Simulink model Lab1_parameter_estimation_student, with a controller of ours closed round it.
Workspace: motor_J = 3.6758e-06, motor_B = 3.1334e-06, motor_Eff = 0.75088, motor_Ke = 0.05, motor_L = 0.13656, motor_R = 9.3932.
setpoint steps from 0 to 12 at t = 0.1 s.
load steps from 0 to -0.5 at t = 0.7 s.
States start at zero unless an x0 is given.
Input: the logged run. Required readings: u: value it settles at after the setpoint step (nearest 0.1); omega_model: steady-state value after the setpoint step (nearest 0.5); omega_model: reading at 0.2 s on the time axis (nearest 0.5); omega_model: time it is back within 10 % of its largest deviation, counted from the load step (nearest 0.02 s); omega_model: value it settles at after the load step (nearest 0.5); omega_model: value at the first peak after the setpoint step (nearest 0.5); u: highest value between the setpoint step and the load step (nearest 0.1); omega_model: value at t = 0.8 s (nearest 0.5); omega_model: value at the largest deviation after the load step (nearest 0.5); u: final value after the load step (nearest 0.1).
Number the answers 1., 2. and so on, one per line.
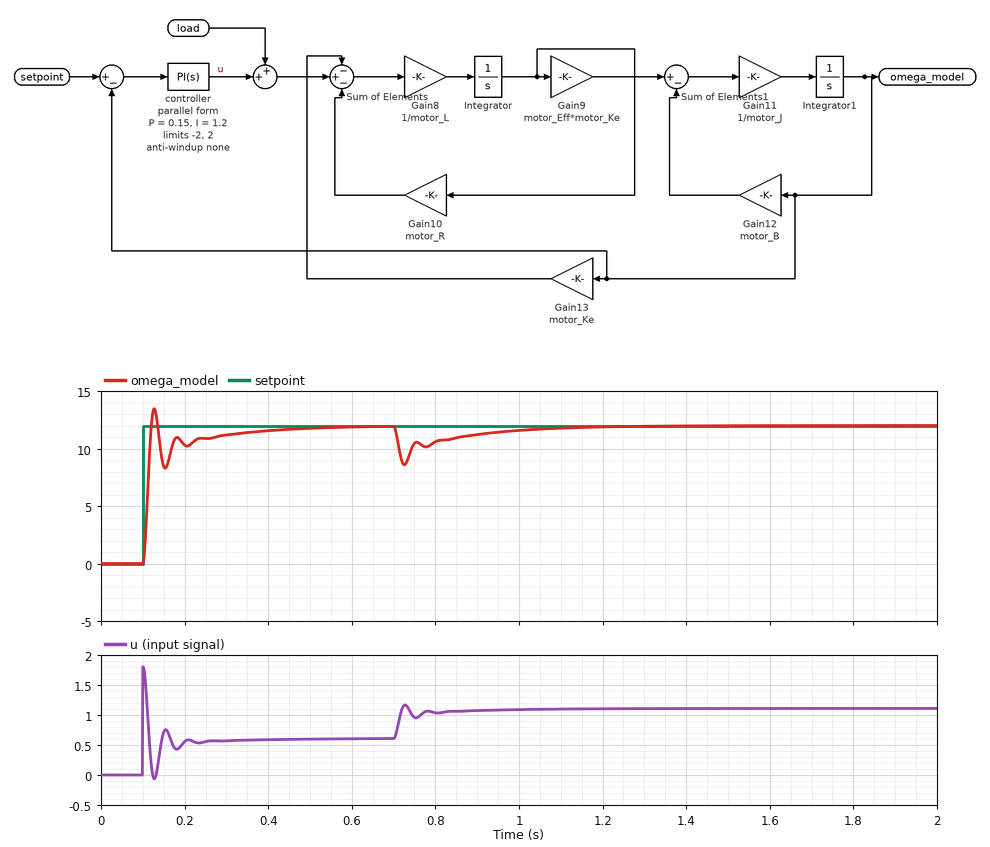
1. 0.6
2. 12.0
3. 10.5
4. 0.34 s
5. 12.0
6. 13.5
7. 1.8
8. 10.5
9. 8.5
10. 1.1
